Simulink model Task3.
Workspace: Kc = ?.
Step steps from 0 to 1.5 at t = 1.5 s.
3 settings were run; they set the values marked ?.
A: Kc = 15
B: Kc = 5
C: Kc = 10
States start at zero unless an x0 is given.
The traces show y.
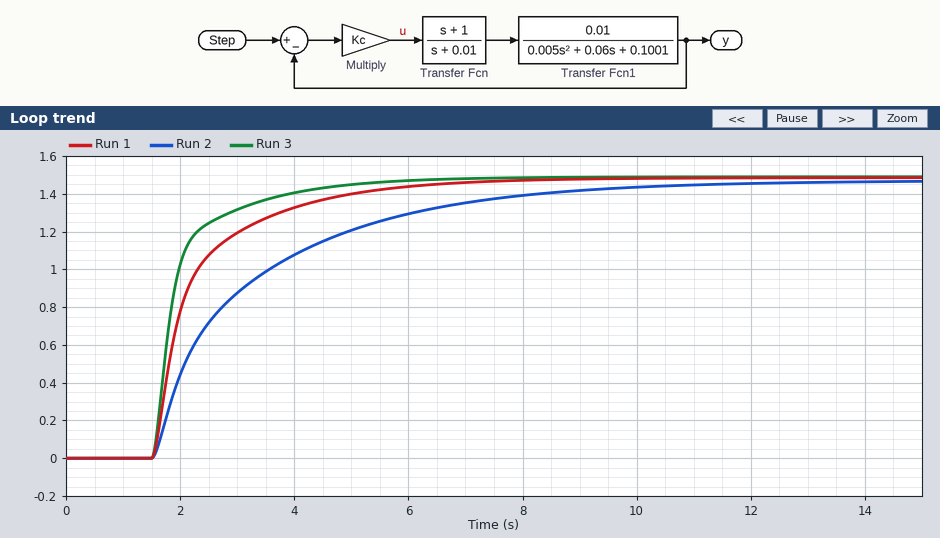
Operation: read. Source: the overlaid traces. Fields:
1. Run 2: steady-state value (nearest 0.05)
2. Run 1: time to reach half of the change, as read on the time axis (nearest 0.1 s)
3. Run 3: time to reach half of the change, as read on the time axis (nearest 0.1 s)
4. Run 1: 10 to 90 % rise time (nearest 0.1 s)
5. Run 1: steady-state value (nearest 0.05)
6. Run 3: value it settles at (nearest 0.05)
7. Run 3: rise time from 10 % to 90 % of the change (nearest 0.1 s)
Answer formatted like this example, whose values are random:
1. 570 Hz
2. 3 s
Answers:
1. 1.45
2. 2.0 s
3. 1.8 s
4. 2.5 s
5. 1.50
6. 1.50
7. 1.6 s
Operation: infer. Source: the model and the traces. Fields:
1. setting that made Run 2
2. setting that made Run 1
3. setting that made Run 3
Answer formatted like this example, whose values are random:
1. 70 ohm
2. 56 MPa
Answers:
1. B
2. C
3. A
